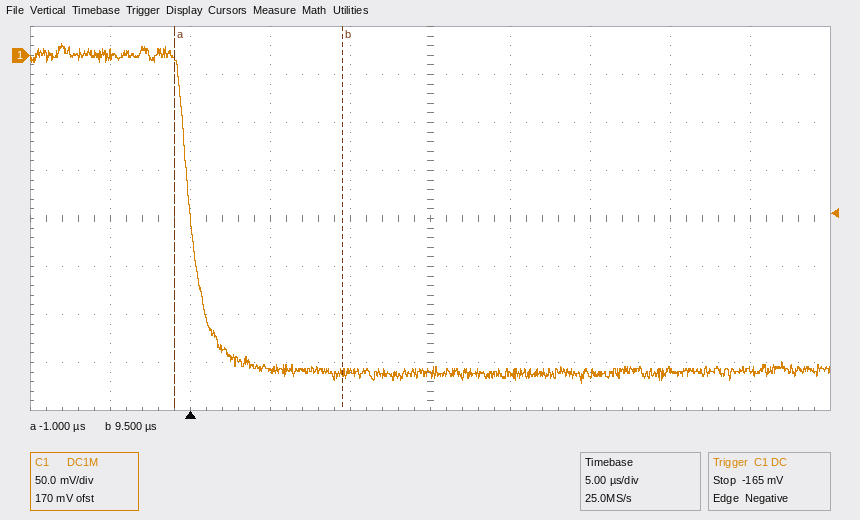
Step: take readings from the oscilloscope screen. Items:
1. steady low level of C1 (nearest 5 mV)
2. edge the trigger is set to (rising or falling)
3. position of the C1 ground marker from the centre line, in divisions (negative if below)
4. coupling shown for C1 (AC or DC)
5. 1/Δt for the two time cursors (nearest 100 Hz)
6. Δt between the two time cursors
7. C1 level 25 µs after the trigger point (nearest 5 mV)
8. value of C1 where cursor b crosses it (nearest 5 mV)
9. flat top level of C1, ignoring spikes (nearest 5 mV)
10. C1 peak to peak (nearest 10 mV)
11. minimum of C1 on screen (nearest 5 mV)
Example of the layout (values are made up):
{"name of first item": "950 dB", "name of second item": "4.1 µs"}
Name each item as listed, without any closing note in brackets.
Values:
{"steady low level of C1": "-330 mV", "edge the trigger is set to": "falling", "position of the C1 ground marker from the centre line, in divisions": "+3.4 div", "coupling shown for C1": "DC", "1/Δt for the two time cursors": "95.2 kHz", "Δt between the two time cursors": "10.5 µs", "C1 level 25 µs after the trigger point": "-330 mV", "value of C1 where cursor b crosses it": "-330 mV", "flat top level of C1, ignoring spikes": "0 mV", "C1 peak to peak": "350 mV", "minimum of C1 on screen": "-340 mV"}
